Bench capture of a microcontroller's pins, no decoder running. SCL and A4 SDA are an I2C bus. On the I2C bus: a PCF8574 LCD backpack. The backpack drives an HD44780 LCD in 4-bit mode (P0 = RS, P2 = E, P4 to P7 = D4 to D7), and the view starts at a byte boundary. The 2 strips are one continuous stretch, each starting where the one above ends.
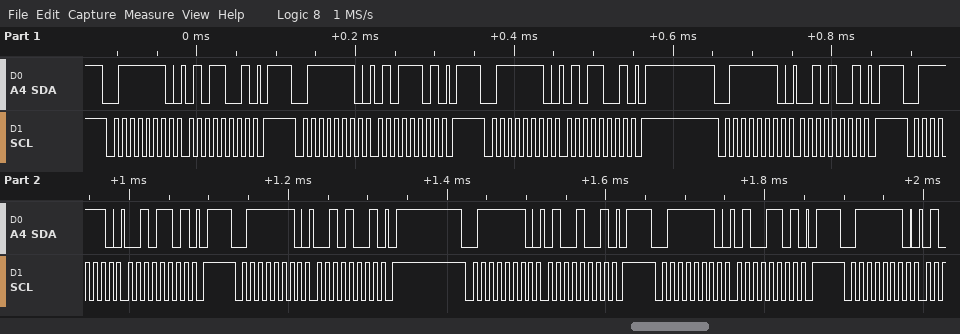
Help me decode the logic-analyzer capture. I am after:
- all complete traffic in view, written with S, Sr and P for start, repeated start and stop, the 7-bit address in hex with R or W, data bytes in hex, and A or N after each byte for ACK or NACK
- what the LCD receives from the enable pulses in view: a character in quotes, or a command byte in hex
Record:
S 3FW A 59 A P S 3FW A 5D A P S 3FW A 59 A P S 3FW A 29 A P S 3FW A 2D A P S 3FW A 29 A P S 3FW A 49 A P S 3FW A 4D A P S 3FW A
'R'
